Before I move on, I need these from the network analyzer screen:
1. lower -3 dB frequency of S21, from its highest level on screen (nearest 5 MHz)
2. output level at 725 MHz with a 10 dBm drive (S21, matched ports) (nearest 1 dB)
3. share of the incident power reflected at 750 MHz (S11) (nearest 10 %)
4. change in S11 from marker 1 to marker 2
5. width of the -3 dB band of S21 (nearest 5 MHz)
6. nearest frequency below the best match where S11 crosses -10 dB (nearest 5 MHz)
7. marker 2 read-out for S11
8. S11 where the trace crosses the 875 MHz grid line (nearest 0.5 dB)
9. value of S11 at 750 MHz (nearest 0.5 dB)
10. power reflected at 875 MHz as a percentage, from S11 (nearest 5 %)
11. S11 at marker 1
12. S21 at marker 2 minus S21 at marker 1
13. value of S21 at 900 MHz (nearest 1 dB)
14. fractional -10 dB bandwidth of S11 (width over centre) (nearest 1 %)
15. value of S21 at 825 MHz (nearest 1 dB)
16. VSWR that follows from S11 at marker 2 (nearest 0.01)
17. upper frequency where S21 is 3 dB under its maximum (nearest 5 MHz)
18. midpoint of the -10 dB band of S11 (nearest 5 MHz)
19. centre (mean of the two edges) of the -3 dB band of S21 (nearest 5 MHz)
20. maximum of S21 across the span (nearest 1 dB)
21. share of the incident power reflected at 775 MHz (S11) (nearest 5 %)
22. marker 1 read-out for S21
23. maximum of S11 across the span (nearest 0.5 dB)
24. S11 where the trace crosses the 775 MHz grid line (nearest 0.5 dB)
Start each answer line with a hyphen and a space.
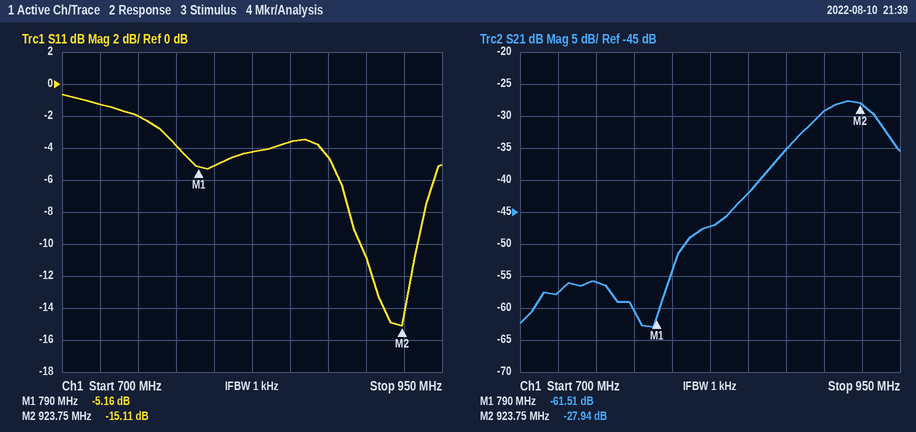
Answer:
- 895 MHz
- -48 dBm
- 60 %
- -9.95 dB
- 40 MHz
- 895 MHz
- -15.11 dB
- -4.5 dB
- -2.0 dB
- 35 %
- -5.16 dB
- 33.57 dB
- -29 dB
- 4 %
- -47 dB
- 1.43
- 935 MHz
- 915 MHz
- 915 MHz
- -28 dB
- 40 %
- -61.51 dB
- -0.5 dB
- -4.0 dB
